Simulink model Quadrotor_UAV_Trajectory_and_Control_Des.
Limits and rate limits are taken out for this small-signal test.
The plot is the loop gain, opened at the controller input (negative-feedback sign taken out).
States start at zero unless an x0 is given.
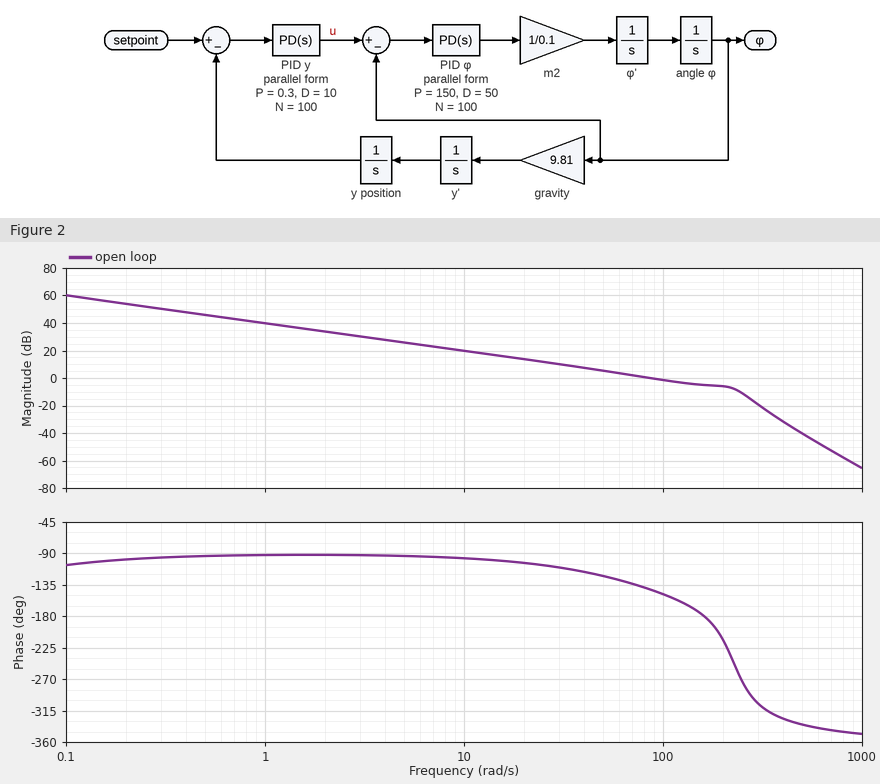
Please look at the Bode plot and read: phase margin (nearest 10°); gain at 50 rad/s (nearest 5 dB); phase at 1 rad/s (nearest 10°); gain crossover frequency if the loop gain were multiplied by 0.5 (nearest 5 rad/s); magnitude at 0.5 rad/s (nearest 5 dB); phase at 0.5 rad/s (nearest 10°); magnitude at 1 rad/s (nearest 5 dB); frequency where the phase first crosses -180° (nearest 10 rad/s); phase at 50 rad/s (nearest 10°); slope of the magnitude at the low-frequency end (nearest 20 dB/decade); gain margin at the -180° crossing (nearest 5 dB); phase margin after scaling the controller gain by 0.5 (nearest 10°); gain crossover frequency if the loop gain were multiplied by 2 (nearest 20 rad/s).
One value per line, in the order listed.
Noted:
40°
5 dB
-90°
45 rad/s
45 dB
-90°
40 dB
160 rad/s
-120°
-20 dB/decade
5 dB
60°
200 rad/s
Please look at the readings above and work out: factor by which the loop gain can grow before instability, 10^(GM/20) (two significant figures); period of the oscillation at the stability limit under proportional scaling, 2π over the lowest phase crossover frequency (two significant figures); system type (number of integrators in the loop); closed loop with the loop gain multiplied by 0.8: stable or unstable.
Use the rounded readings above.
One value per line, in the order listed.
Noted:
1.8
0.039 s
1
stable
